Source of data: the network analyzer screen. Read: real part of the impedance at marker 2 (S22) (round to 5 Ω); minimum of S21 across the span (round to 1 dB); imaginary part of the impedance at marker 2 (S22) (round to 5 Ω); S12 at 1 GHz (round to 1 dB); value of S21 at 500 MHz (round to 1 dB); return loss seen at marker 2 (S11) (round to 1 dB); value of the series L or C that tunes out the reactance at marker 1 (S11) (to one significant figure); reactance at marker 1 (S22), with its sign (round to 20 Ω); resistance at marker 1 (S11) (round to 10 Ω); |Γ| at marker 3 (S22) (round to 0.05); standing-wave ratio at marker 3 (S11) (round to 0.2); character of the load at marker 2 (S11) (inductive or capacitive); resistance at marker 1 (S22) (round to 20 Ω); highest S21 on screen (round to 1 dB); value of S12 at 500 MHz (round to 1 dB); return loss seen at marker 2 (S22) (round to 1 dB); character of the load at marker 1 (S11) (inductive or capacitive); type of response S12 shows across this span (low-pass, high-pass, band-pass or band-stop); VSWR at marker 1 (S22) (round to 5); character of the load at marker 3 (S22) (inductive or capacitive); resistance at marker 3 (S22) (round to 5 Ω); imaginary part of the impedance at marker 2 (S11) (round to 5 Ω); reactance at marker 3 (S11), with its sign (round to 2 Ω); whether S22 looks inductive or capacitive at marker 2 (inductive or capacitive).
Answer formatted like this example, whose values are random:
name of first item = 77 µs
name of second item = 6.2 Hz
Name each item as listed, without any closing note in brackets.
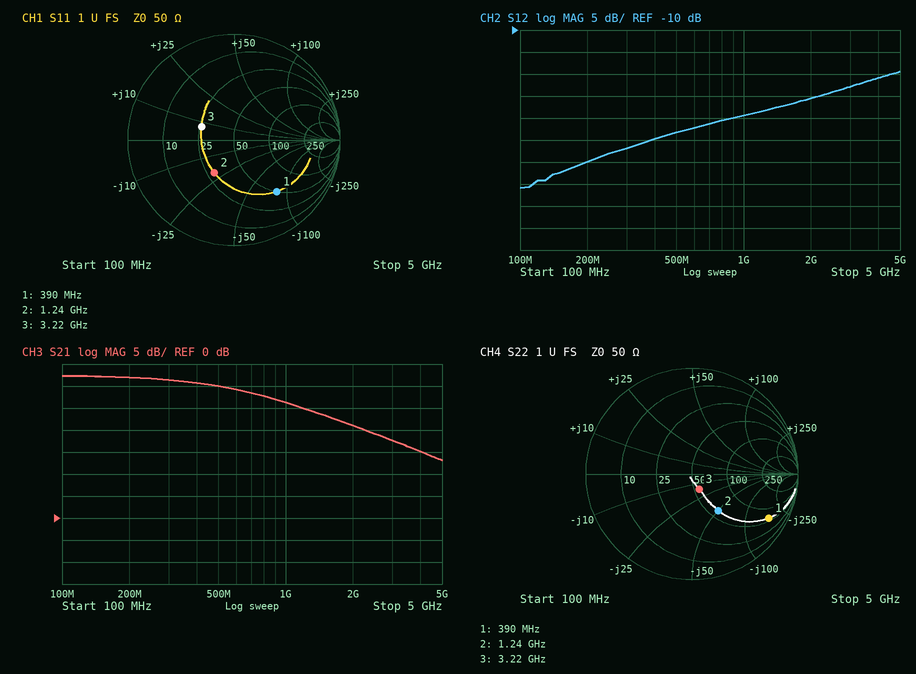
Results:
real part of the impedance at marker 2 (S22) = 60 Ω
minimum of S21 across the span = 13 dB
imaginary part of the impedance at marker 2 (S22) = -50 Ω
S12 at 1 GHz = -29 dB
value of S21 at 500 MHz = 30 dB
return loss seen at marker 2 (S11) = 9 dB
value of the series L or C that tunes out the reactance at marker 1 (S11) = 30 nH
reactance at marker 1 (S22), with its sign = -160 Ω
resistance at marker 1 (S11) = 50 Ω
|Γ| at marker 3 (S22) = 0.15
standing-wave ratio at marker 3 (S11) = 2.0
character of the load at marker 2 (S11) = capacitive
resistance at marker 1 (S22) = 60 Ω
highest S21 on screen = 32 dB
value of S12 at 500 MHz = -33 dB
return loss seen at marker 2 (S22) = 7 dB
character of the load at marker 1 (S11) = capacitive
type of response S12 shows across this span = high-pass
VSWR at marker 1 (S22) = 10
character of the load at marker 3 (S22) = capacitive
resistance at marker 3 (S22) = 55 Ω
imaginary part of the impedance at marker 2 (S11) = -20 Ω
reactance at marker 3 (S11), with its sign = +8 Ω
whether S22 looks inductive or capacitive at marker 2 = capacitive
